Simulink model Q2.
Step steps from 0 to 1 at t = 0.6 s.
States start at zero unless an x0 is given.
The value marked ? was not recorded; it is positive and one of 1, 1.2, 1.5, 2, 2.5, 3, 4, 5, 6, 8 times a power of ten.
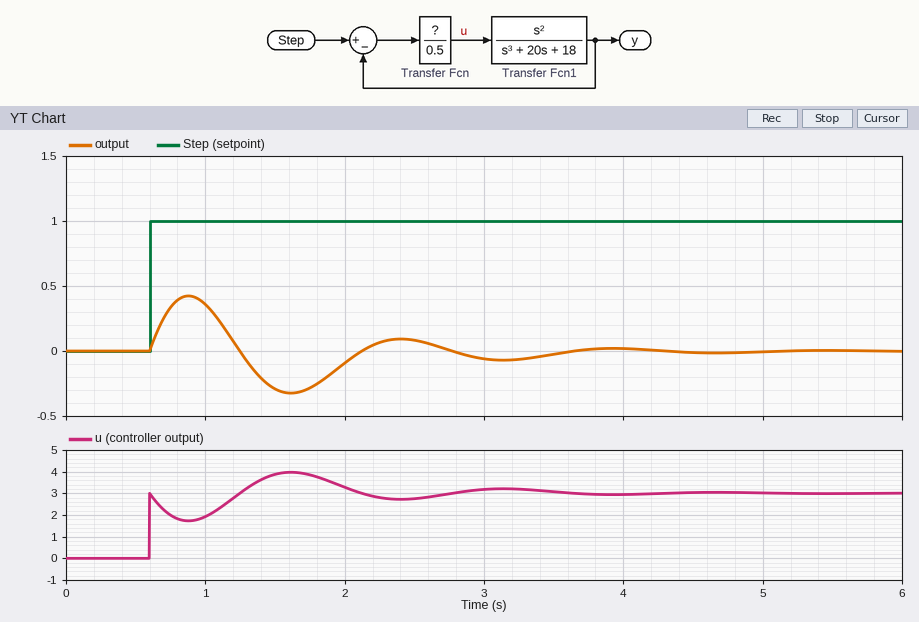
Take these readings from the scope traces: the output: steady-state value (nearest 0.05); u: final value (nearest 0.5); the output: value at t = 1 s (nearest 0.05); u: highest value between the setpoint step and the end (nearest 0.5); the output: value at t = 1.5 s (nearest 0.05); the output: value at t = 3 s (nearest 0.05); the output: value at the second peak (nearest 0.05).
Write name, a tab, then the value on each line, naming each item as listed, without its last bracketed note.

the output: steady-state value	0.00
u: final value	3.0
the output: value at t = 1 s	0.35
u: highest value between the setpoint step and the end	4.0
the output: value at t = 1.5 s	-0.30
the output: value at t = 3 s	-0.05
the output: value at the second peak	0.10
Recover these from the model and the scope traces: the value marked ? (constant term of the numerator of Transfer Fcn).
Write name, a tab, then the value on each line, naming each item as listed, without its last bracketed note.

the value marked ?	1.5
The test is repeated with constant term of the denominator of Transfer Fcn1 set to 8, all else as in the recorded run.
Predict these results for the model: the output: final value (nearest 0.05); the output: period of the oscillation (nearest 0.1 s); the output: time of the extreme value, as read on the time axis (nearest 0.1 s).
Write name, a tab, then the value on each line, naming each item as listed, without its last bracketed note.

the output: final value	0.00
the output: period of the oscillation	1.5 s
the output: time of the extreme value, as read on the time axis	0.9 s
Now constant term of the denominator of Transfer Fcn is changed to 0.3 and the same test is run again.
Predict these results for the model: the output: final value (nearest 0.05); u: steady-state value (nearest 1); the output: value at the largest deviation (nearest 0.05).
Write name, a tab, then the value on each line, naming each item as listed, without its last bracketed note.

the output: final value	0.00
u: steady-state value	5
the output: value at the largest deviation	0.55
